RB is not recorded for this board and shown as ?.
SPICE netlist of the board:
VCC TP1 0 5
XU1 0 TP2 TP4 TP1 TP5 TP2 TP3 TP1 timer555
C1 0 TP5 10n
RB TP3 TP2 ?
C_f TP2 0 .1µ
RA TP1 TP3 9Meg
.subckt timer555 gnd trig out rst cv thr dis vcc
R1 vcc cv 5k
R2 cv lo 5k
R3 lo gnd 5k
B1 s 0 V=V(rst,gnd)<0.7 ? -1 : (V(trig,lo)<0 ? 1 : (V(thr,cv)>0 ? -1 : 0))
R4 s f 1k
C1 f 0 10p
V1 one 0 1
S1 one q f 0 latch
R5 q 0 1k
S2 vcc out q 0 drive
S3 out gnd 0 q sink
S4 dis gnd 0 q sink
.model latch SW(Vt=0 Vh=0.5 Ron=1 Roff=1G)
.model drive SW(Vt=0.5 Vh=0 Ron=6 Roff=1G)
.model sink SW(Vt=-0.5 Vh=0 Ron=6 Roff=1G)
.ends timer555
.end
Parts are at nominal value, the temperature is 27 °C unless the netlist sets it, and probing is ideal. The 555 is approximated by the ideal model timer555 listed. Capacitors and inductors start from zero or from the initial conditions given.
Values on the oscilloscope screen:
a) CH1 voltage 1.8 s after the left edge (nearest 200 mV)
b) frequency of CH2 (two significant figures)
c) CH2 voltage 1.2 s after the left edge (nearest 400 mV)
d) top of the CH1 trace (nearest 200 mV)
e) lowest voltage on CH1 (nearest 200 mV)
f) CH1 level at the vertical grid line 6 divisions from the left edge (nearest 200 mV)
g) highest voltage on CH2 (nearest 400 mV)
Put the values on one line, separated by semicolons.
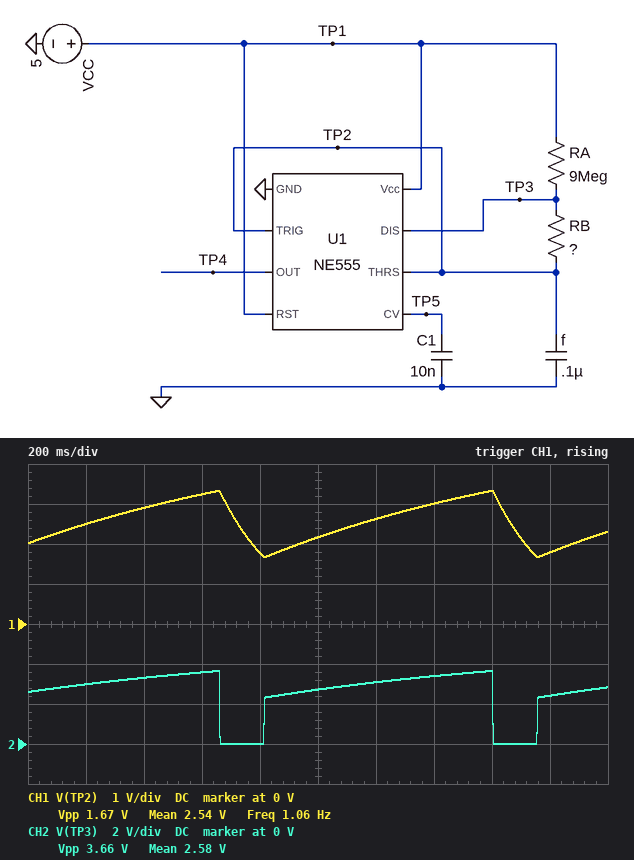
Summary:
1.8 V; 1.1 Hz; 3.2 V; 3.4 V; 1.6 V; 2.6 V; 3.6 V
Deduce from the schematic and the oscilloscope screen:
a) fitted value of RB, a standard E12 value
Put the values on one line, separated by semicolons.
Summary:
2.2 MΩ
